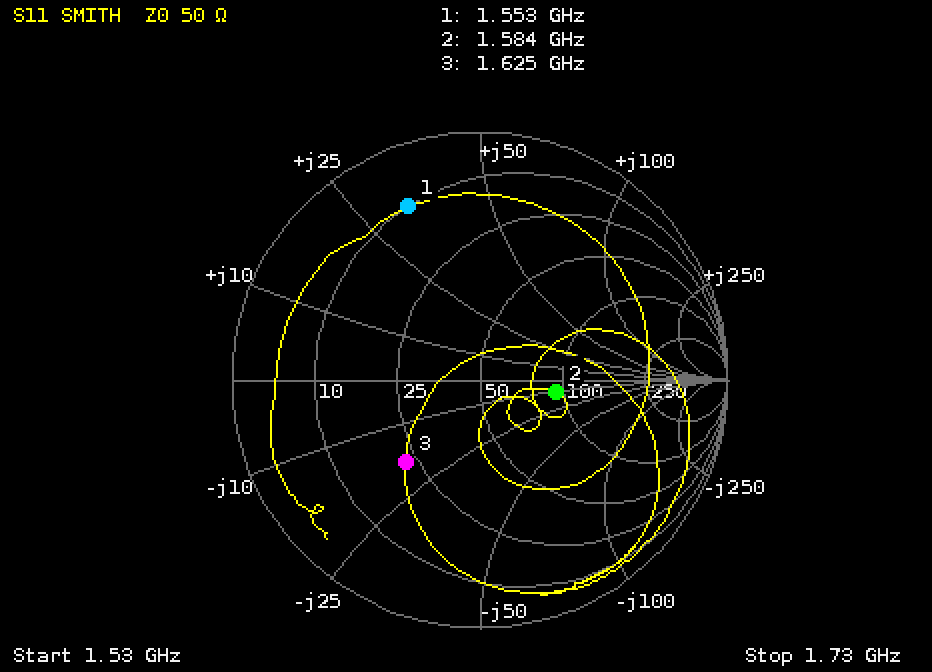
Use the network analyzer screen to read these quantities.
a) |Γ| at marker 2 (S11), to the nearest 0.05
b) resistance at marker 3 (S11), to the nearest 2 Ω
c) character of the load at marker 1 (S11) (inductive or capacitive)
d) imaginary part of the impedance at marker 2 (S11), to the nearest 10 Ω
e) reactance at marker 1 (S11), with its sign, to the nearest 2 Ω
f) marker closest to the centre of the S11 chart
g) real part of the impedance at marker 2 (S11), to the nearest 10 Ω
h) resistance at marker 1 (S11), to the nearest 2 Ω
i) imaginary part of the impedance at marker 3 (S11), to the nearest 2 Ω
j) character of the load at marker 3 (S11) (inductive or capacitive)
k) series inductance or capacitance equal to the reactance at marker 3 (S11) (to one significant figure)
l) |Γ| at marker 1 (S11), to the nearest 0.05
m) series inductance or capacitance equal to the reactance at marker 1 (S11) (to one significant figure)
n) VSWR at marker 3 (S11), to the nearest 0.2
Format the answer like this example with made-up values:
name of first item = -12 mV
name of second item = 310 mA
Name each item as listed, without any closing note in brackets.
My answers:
|Γ| at marker 2 (S11), to the nearest 0.05 = 0.30
resistance at marker 3 (S11), to the nearest 2 Ω = 22 Ω
character of the load at marker 1 (S11) = inductive
imaginary part of the impedance at marker 2 (S11), to the nearest 10 Ω = -10 Ω
reactance at marker 1 (S11), with its sign, to the nearest 2 Ω = +32 Ω
marker closest to the centre of the S11 chart = marker 2
real part of the impedance at marker 2 (S11), to the nearest 10 Ω = 90 Ω
resistance at marker 1 (S11), to the nearest 2 Ω = 10 Ω
imaginary part of the impedance at marker 3 (S11), to the nearest 2 Ω = -18 Ω
character of the load at marker 3 (S11) = capacitive
series inductance or capacitance equal to the reactance at marker 3 (S11) = 5 pF
|Γ| at marker 1 (S11), to the nearest 0.05 = 0.75
series inductance or capacitance equal to the reactance at marker 1 (S11) = 3 nH
VSWR at marker 3 (S11), to the nearest 0.2 = 2.6
